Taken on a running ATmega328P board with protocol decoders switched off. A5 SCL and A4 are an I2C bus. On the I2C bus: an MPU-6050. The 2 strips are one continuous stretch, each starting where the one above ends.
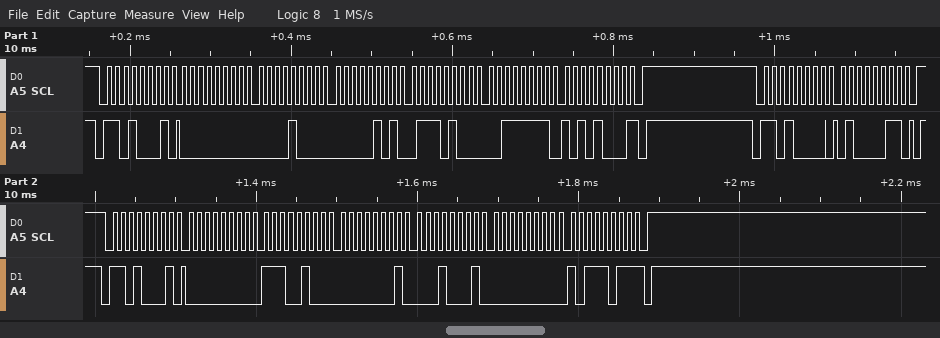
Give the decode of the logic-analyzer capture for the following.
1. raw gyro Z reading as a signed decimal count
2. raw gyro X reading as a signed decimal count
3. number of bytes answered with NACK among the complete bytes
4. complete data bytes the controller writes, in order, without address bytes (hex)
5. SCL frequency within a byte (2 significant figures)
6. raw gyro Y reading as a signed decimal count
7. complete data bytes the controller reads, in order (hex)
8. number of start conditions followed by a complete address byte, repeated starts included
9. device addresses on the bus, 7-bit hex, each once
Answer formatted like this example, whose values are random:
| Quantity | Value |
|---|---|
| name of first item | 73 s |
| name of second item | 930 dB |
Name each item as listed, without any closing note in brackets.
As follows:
| Quantity | Value |
|---|---|
| raw gyro Z reading as a signed decimal count | 187 |
| raw gyro X reading as a signed decimal count | 228 |
| number of bytes answered with NACK among the complete bytes | 2 |
| complete data bytes the controller writes, in order, without address bytes | 43 |
| SCL frequency within a byte | 100 kHz |
| raw gyro Y reading as a signed decimal count | 273 |
| complete data bytes the controller reads, in order | 00 08 05 74 3F A8 00 E4 01 11 00 BB |
| number of start conditions followed by a complete address byte, repeated starts included | 3 |
| device addresses on the bus, 7-bit hex, each once | 0x68 |
